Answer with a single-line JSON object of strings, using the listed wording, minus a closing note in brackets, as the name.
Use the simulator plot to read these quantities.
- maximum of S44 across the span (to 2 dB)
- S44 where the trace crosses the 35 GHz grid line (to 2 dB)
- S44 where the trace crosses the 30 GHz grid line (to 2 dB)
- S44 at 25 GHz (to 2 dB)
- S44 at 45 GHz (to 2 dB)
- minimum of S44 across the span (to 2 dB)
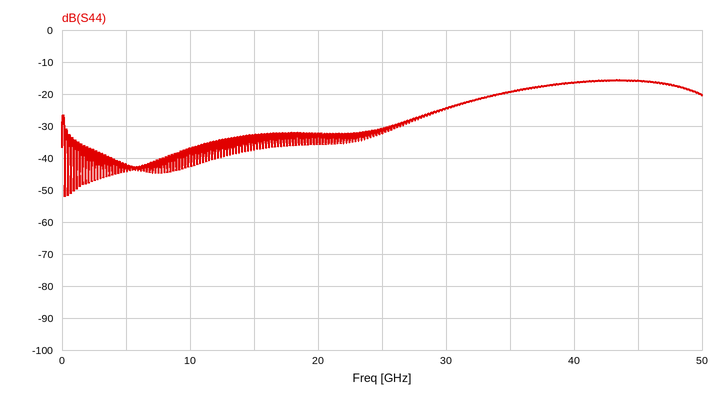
{"maximum of S44 across the span": "-16 dB", "S44 where the trace crosses the 35 GHz grid line": "-20 dB", "S44 where the trace crosses the 30 GHz grid line": "-24 dB", "S44 at 25 GHz": "-32 dB", "S44 at 45 GHz": "-16 dB", "minimum of S44 across the span": "-52 dB"}
